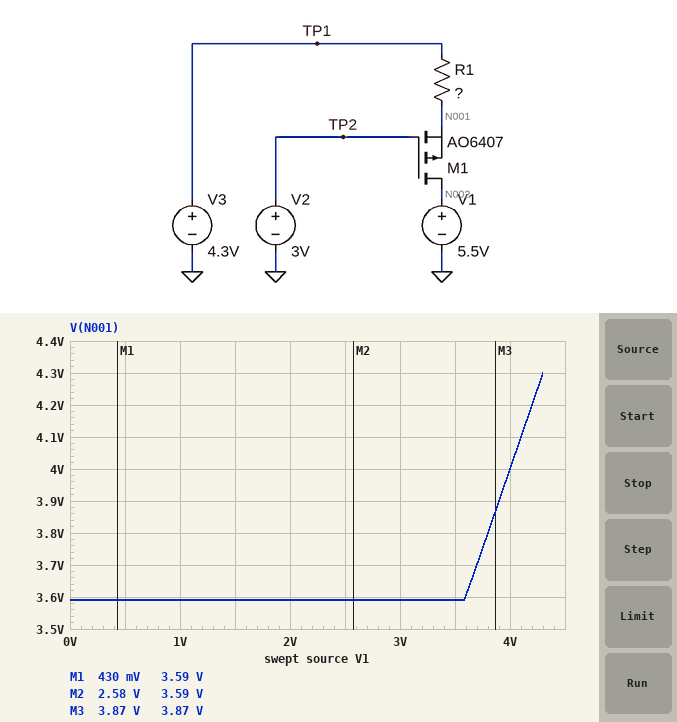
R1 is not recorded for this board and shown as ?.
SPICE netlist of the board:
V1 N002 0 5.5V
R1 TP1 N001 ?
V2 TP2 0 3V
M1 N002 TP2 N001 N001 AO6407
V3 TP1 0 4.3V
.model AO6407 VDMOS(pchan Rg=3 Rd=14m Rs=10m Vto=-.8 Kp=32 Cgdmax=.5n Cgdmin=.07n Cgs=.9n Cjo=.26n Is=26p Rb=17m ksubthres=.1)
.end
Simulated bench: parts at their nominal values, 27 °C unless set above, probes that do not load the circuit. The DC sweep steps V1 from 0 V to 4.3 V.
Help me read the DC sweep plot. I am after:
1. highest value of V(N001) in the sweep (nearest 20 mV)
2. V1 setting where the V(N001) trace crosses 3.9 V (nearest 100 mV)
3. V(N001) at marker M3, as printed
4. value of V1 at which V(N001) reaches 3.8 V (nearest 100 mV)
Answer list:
4.30 V
3.9 V
3.87 V
3.8 V
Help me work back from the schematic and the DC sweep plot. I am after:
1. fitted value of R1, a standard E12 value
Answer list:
330 Ω
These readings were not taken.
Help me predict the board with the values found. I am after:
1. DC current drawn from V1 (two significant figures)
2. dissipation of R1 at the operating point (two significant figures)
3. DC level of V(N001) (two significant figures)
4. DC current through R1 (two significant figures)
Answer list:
3.6 mA
4.4 mW
5.5 V
3.6 mA
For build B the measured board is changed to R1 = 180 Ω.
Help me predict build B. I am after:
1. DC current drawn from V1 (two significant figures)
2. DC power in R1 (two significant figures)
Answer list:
6.7 mA
8.0 mW
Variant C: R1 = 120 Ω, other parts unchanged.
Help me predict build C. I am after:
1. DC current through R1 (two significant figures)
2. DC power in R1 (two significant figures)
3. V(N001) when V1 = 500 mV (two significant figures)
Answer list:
10 mA
12 mW
3.6 V
